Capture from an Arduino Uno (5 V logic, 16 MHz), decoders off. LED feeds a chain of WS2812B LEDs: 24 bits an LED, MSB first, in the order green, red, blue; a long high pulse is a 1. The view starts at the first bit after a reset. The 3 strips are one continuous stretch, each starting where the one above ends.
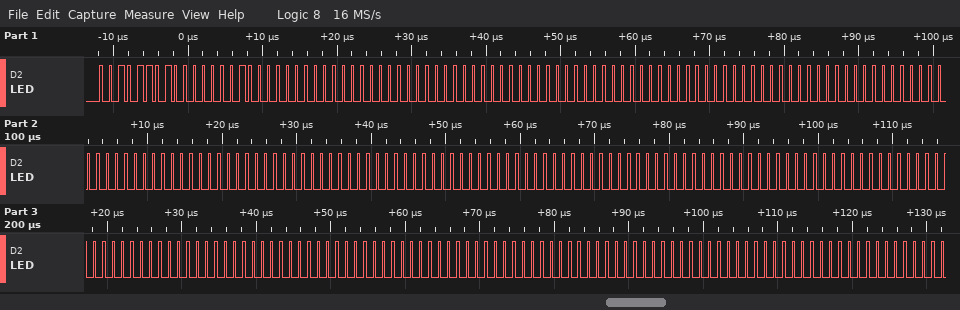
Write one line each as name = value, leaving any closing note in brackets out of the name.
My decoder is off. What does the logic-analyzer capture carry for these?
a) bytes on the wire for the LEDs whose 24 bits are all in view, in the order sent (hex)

bytes on the wire for the LEDs whose 24 bits are all in view, in the order sent = 2D 01 00 00 00 00 00 00 00 00 00 00 00 00 00 00 00 00 00 00 00 00 00 00 00 00 00 00 00 00 00 00 00
